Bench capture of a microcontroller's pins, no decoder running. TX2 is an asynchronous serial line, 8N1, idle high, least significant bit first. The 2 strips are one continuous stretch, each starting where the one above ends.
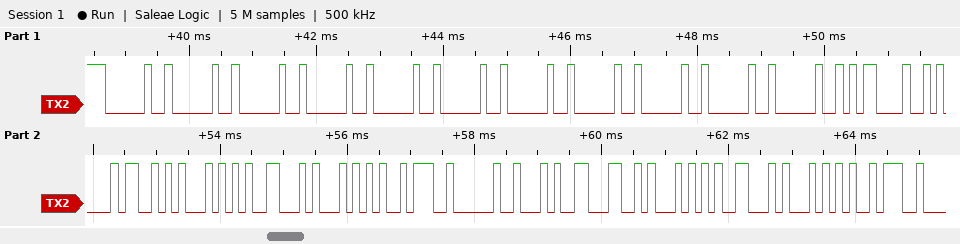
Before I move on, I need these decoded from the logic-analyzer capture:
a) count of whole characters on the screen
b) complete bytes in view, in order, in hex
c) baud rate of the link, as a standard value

25
20 20 20 20 20 20 20 20 20 20 20 0D 0A 53 54 46 54 3A 20 94 4C 54 46 54 3A
9600 baud
